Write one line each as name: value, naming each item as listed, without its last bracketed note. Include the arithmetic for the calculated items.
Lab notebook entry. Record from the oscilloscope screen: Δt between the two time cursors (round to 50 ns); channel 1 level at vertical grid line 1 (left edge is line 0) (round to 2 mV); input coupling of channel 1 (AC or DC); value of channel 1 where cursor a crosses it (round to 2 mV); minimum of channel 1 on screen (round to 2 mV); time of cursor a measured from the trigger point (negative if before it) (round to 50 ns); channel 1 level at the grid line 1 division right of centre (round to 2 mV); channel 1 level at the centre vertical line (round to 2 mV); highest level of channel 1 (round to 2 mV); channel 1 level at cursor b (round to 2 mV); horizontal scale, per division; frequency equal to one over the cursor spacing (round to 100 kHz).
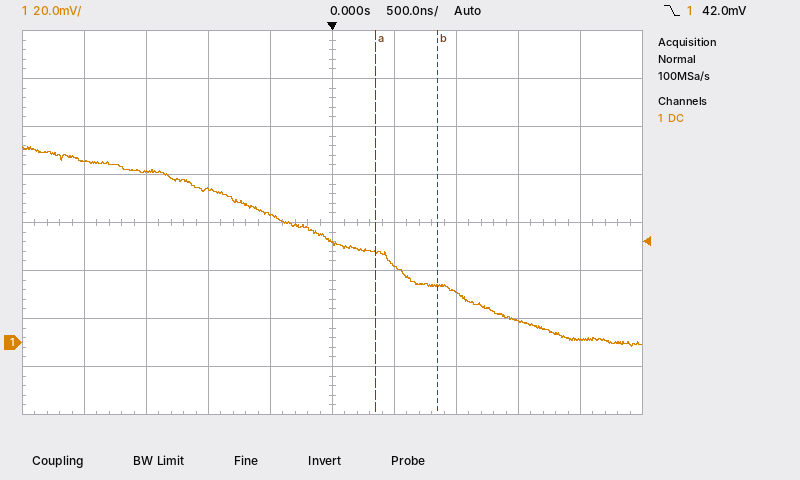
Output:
Δt between the two time cursors: 500 ns
channel 1 level at vertical grid line 1 (left edge is line 0): 76 mV
input coupling of channel 1: DC
value of channel 1 where cursor a crosses it: 38 mV
minimum of channel 1 on screen: -2 mV
time of cursor a measured from the trigger point (negative if before it): +350 ns
channel 1 level at the grid line 1 division right of centre: 32 mV
channel 1 level at the centre vertical line: 42 mV
highest level of channel 1: 82 mV
channel 1 level at cursor b: 24 mV
horizontal scale, per division: 500 ns
frequency equal to one over the cursor spacing: 1 / 500 ns ≈ 2.0 MHz
